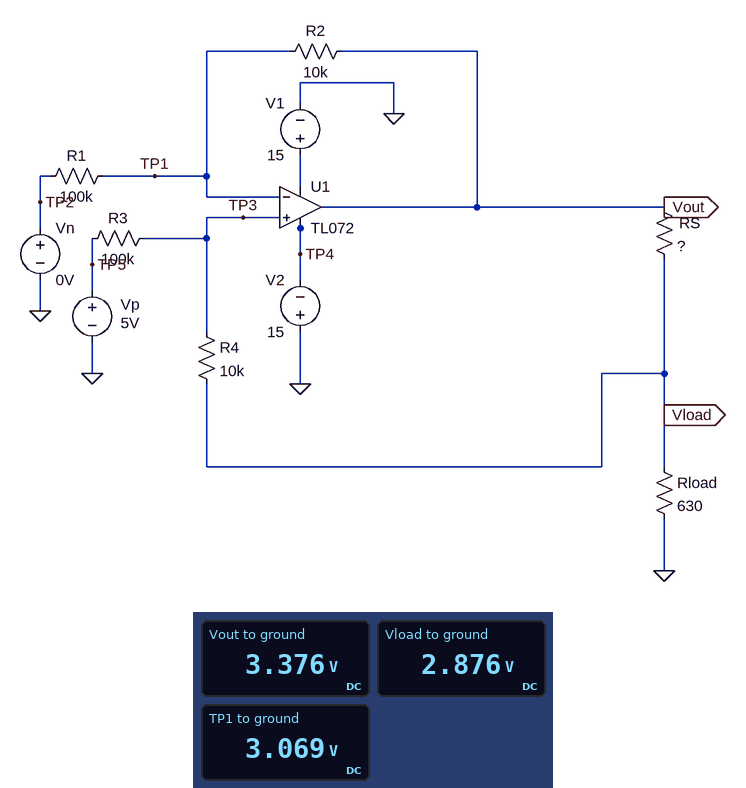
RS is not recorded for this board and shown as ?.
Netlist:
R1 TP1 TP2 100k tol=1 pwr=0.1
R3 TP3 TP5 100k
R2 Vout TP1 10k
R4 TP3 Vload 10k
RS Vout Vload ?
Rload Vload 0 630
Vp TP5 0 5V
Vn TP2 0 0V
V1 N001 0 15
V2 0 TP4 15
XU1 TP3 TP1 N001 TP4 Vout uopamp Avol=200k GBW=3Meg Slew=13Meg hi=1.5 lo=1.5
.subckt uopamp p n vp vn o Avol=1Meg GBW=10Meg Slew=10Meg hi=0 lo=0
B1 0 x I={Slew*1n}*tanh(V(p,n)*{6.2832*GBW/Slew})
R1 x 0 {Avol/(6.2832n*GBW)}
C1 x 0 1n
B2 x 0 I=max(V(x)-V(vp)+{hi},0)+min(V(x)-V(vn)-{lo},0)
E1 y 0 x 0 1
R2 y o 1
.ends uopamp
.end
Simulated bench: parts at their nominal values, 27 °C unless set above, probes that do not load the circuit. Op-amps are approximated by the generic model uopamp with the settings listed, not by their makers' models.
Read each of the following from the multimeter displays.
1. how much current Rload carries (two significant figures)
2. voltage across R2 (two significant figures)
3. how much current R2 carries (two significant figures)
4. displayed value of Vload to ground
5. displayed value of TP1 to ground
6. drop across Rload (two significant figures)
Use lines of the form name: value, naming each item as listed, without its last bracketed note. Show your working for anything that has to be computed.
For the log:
how much current Rload carries: (2.876 V) / 630 Ω = 4.6 mA
voltage across R2: 3.376 V - 3.069 V = 310 mV
how much current R2 carries: (3.376 V - 3.069 V) / 10 kΩ = 31 µA
displayed value of Vload to ground: 2.876 V
displayed value of TP1 to ground: 3.069 V
drop across Rload: 2.876 V = 2.9 V
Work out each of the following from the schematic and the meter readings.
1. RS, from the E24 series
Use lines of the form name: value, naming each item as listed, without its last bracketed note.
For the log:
RS, from the E24 series: 110 Ω
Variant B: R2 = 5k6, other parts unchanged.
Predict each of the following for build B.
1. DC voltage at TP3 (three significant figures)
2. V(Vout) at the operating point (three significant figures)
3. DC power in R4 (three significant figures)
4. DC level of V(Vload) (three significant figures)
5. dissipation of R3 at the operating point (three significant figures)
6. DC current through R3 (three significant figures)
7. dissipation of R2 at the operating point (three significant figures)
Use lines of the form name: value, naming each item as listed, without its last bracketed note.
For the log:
DC voltage at TP3: 2.50 V
V(Vout) at the operating point: 2.64 V
DC power in R4: 6.25 µW
DC level of V(Vload): 2.25 V
dissipation of R3 at the operating point: 62.5 µW
DC current through R3: 25.0 µA
dissipation of R2 at the operating point: 3.50 µW
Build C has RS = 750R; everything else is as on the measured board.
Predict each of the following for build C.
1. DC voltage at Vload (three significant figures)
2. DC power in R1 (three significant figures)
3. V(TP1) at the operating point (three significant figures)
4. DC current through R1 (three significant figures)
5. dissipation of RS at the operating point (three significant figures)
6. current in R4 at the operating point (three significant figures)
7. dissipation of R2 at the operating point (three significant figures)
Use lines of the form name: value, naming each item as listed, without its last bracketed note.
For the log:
DC voltage at Vload: 446 mV
DC power in R1: 7.40 µW
V(TP1) at the operating point: 860 mV
DC current through R1: 8.60 µA
dissipation of RS at the operating point: 333 µW
current in R4 at the operating point: 41.4 µA
dissipation of R2 at the operating point: 740 nW
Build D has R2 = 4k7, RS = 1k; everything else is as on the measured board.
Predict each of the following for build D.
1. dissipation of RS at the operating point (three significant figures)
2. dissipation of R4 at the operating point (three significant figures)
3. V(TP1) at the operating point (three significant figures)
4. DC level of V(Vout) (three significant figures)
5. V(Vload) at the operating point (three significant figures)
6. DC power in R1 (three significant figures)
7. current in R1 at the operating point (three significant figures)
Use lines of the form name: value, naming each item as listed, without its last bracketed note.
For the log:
dissipation of RS at the operating point: 212 µW
dissipation of R4 at the operating point: 18.1 µW
V(TP1) at the operating point: 743 mV
DC level of V(Vout): 778 mV
V(Vload) at the operating point: 317 mV
DC power in R1: 5.52 µW
current in R1 at the operating point: 7.43 µA
